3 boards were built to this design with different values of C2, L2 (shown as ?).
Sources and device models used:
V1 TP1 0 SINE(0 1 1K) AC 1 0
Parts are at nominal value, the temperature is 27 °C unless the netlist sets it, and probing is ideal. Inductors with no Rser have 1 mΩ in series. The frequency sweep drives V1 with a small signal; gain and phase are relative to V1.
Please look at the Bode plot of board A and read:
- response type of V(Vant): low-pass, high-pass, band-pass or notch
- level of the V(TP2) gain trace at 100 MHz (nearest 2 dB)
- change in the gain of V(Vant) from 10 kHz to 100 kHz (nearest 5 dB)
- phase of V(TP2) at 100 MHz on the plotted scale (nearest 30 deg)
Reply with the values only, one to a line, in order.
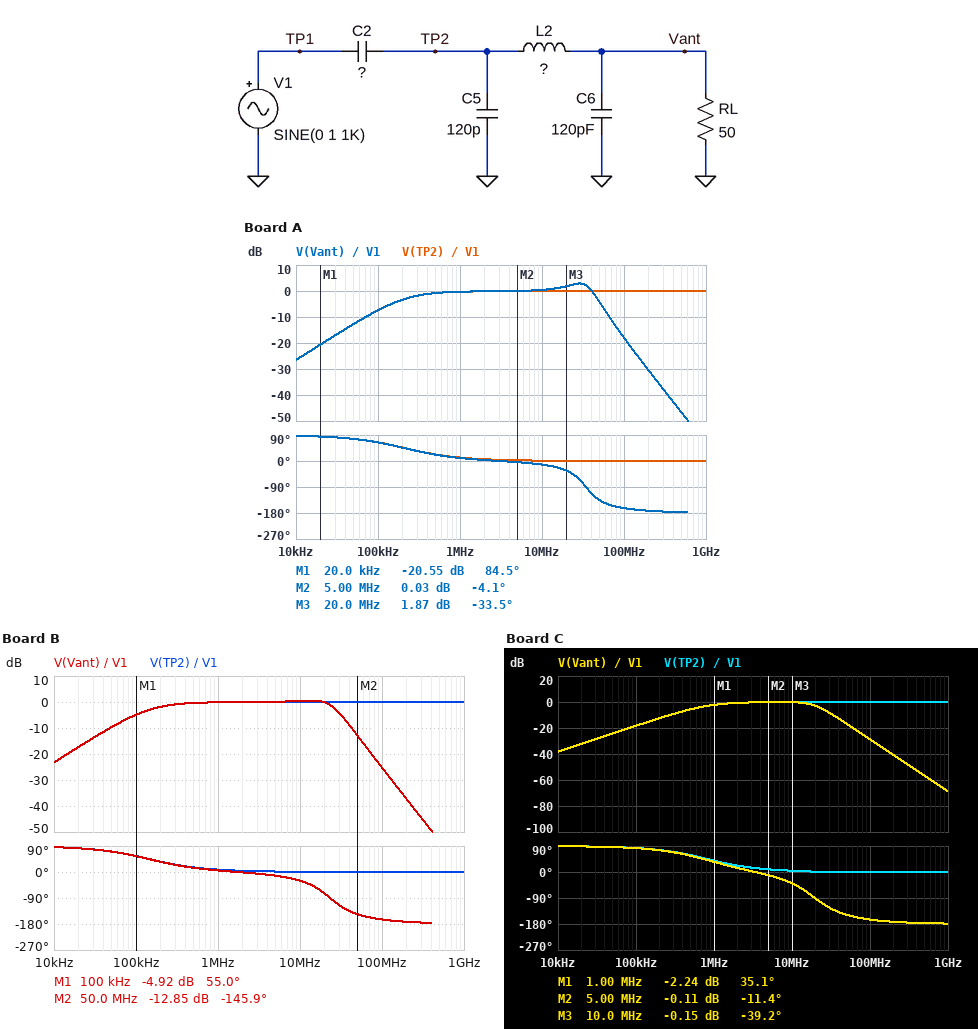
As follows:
band-pass
0 dB
20 dB
0 deg
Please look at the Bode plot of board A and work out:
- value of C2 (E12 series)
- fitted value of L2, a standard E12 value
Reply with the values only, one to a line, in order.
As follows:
15 nF
180 nH
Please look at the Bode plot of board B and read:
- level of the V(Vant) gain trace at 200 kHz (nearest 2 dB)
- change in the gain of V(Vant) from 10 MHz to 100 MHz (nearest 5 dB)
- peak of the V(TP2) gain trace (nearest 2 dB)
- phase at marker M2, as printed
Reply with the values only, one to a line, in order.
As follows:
-2 dB
-25 dB
0 dB
-145.9 deg
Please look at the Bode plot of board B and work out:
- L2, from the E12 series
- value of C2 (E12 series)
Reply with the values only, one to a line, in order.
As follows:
390 nH
22 nF
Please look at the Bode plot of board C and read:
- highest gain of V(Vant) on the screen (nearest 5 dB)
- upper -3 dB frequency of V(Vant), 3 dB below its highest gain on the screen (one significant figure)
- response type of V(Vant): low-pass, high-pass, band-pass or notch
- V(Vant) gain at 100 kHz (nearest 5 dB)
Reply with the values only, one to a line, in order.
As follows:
0 dB
20 MHz
band-pass
-20 dB
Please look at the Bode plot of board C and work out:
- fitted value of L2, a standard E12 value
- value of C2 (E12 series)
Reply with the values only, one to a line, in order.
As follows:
560 nH
3.9 nF
